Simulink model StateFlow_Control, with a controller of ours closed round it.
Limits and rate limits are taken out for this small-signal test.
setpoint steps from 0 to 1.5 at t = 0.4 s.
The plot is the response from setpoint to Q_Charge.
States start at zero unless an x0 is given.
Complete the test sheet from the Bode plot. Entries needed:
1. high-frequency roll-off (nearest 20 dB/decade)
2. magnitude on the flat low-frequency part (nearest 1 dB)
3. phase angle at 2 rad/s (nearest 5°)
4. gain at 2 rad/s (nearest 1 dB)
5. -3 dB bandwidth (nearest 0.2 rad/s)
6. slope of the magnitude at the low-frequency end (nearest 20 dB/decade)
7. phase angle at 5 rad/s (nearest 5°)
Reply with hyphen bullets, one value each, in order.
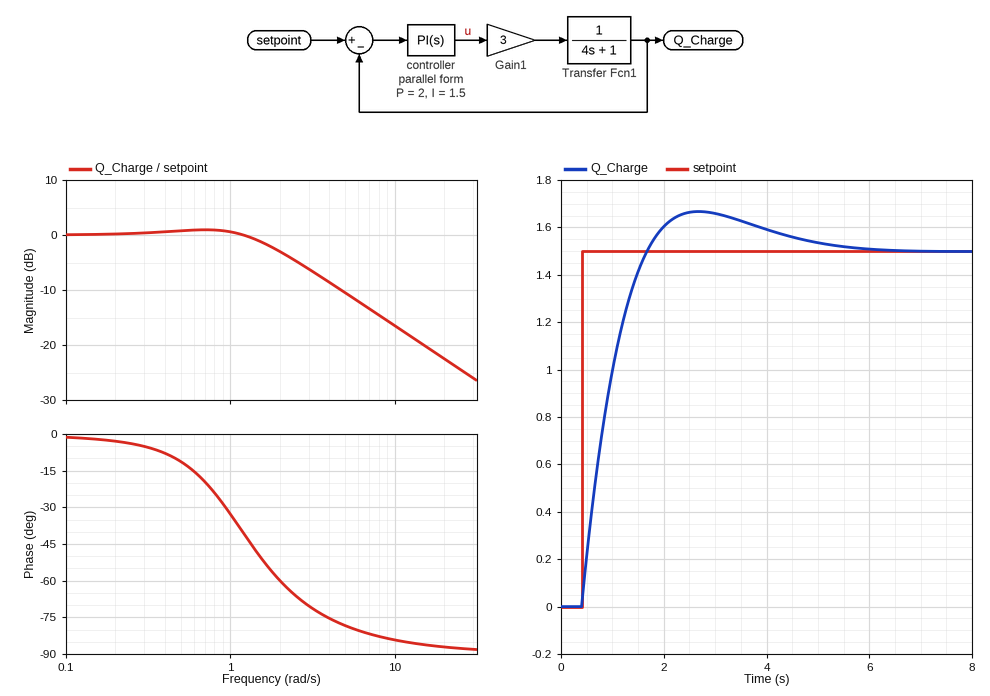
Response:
- -20 dB/decade
- 0 dB
- -60°
- -3 dB
- 2.0 rad/s
- 0 dB/decade
- -80°
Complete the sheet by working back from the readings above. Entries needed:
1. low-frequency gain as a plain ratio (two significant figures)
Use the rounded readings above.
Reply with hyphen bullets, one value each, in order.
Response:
- 1.0
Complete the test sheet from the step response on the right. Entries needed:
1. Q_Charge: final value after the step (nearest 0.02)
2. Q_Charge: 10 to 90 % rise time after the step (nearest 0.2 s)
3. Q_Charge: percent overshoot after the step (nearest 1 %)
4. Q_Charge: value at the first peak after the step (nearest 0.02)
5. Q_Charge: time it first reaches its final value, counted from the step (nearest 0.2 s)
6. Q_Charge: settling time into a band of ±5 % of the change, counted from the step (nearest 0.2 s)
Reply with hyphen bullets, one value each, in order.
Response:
- 1.50
- 1.0 s
- 11 %
- 1.66
- 1.2 s
- 3.8 s
